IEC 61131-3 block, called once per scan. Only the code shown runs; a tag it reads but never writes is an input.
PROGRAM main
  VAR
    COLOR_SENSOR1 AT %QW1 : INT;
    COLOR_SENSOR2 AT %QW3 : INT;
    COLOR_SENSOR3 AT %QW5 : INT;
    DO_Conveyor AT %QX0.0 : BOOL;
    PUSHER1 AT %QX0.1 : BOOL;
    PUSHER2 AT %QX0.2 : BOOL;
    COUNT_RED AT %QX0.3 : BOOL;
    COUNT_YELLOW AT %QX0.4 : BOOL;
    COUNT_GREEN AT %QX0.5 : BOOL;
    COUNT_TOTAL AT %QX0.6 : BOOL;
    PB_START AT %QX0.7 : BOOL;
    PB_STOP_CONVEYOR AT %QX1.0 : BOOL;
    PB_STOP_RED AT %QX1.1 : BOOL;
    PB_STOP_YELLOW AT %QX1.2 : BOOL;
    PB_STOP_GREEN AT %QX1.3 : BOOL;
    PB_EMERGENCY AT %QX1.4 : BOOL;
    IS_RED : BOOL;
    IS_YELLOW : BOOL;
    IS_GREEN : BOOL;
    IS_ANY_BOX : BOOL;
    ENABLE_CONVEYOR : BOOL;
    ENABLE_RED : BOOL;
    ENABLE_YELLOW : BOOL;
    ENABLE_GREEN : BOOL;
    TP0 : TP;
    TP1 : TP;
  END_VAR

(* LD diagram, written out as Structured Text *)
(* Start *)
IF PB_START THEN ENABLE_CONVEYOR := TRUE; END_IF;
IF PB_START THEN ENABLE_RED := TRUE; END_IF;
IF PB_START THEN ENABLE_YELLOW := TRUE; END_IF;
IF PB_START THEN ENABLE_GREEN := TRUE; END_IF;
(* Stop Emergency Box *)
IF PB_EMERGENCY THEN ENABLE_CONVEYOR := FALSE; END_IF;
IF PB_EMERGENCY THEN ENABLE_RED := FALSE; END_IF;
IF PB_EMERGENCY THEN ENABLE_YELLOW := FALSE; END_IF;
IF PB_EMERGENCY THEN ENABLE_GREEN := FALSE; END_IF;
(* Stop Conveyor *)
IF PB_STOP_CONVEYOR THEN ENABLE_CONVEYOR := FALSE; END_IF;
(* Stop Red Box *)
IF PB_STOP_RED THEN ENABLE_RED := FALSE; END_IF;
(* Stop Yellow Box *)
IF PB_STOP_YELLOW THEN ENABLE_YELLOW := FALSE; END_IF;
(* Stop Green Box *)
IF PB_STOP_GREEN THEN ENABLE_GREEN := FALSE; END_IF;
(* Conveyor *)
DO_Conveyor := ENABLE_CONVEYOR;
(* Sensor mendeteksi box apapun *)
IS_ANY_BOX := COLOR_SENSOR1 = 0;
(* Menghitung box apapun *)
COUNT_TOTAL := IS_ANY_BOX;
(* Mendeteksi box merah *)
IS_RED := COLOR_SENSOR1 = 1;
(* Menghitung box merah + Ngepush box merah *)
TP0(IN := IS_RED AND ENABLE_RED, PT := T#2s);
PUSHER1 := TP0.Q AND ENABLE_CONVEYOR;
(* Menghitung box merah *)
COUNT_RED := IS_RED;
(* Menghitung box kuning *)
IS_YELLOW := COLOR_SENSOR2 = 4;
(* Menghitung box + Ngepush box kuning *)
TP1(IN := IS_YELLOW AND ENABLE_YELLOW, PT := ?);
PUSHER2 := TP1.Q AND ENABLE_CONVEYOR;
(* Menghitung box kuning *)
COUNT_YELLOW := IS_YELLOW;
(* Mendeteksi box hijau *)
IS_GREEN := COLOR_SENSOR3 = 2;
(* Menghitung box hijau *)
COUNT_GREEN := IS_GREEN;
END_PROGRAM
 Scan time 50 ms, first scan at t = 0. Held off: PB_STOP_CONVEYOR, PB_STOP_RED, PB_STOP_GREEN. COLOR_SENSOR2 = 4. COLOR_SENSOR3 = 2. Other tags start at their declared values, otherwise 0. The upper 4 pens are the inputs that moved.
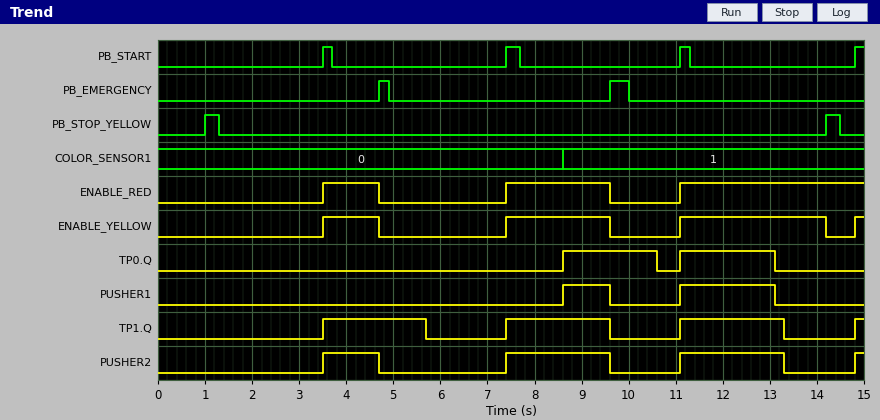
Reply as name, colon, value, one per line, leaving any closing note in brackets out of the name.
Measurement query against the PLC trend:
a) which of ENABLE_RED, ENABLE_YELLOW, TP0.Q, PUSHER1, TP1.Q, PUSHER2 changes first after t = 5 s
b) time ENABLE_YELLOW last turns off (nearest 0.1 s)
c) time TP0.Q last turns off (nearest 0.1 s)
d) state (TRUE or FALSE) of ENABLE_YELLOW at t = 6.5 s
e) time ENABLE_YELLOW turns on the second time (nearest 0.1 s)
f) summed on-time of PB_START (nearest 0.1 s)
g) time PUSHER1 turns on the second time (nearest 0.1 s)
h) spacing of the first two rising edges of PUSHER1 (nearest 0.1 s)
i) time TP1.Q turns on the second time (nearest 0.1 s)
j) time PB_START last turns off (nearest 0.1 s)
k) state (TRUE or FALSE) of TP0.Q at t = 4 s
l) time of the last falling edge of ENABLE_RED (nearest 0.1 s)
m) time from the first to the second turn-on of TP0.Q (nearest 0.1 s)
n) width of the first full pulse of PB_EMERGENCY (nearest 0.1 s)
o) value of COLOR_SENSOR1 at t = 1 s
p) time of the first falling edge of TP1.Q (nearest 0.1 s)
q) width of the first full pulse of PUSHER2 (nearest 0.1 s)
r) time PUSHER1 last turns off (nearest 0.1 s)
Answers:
which of ENABLE_RED, ENABLE_YELLOW, TP0.Q, PUSHER1, TP1.Q, PUSHER2 changes first after t = 5 s: TP1.Q
time ENABLE_YELLOW last turns off: 14.2 s
time TP0.Q last turns off: 13.1 s
state (TRUE or FALSE) of ENABLE_YELLOW at t = 6.5 s: FALSE
time ENABLE_YELLOW turns on the second time: 7.4 s
summed on-time of PB_START: 0.9 s
time PUSHER1 turns on the second time: 11.1 s
spacing of the first two rising edges of PUSHER1: 2.5 s
time TP1.Q turns on the second time: 7.4 s
time PB_START last turns off: 11.3 s
state (TRUE or FALSE) of TP0.Q at t = 4 s: FALSE
time of the last falling edge of ENABLE_RED: 9.6 s
time from the first to the second turn-on of TP0.Q: 2.5 s
width of the first full pulse of PB_EMERGENCY: 0.2 s
value of COLOR_SENSOR1 at t = 1 s: 0
time of the first falling edge of TP1.Q: 5.7 s
width of the first full pulse of PUSHER2: 1.2 s
time PUSHER1 last turns off: 13.1 s
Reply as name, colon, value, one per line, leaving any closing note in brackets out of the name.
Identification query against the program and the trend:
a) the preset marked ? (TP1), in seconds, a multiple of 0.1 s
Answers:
the preset marked ? (TP1), in seconds, a multiple of 0.1 s: 2.2 s
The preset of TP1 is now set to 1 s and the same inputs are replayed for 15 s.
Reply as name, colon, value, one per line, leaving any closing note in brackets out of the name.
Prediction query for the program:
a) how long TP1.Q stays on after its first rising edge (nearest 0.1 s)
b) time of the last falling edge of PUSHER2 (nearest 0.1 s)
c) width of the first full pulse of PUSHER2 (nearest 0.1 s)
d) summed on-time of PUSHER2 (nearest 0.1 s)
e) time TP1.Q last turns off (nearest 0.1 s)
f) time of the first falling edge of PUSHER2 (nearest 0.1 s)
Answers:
how long TP1.Q stays on after its first rising edge: 1.0 s
time of the last falling edge of PUSHER2: 12.1 s
width of the first full pulse of PUSHER2: 1.0 s
summed on-time of PUSHER2: 3.2 s
time TP1.Q last turns off: 12.1 s
time of the first falling edge of PUSHER2: 4.5 s
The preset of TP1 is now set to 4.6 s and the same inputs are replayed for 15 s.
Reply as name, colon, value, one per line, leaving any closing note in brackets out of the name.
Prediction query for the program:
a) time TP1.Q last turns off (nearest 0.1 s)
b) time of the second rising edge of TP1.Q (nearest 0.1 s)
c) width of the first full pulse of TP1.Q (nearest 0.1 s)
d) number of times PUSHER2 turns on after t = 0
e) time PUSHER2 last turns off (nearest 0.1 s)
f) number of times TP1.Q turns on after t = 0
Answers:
time TP1.Q last turns off: 8.1 s
time of the second rising edge of TP1.Q: 11.1 s
width of the first full pulse of TP1.Q: 4.6 s
number of times PUSHER2 turns on after t = 0: 3
time PUSHER2 last turns off: 8.1 s
number of times TP1.Q turns on after t = 0: 2
